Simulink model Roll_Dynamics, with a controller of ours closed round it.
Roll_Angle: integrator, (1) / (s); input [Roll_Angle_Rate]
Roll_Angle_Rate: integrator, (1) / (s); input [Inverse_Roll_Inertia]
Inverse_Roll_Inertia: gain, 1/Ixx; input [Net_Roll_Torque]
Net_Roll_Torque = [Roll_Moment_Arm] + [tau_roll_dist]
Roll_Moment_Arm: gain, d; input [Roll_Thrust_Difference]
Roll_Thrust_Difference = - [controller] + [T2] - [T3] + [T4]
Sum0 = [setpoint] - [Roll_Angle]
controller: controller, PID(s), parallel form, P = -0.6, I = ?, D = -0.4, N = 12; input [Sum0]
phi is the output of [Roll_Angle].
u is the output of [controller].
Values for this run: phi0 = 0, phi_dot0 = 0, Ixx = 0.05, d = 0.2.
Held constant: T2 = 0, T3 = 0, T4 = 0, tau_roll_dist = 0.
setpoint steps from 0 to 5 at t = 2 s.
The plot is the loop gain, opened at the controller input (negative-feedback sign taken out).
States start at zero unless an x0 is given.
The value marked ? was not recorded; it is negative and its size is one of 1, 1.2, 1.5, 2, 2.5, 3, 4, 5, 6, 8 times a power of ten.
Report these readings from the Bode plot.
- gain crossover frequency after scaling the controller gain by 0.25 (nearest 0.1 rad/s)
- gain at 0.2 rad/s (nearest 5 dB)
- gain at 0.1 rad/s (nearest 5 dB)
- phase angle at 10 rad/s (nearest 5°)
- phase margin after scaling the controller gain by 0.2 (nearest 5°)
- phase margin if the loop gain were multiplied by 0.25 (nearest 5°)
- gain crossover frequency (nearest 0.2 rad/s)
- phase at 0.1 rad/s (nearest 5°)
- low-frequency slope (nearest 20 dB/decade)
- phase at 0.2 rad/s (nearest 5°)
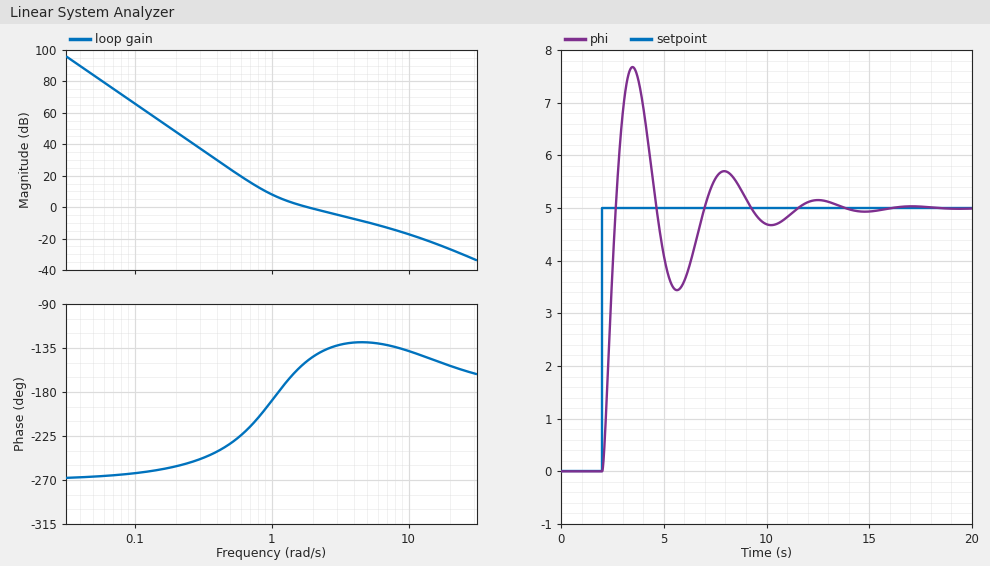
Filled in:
0.8 rad/s
50 dB
65 dB
-140°
-30°
-25°
1.8 rad/s
-265°
-60 dB/decade
-255°
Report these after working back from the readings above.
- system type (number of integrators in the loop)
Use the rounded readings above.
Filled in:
3
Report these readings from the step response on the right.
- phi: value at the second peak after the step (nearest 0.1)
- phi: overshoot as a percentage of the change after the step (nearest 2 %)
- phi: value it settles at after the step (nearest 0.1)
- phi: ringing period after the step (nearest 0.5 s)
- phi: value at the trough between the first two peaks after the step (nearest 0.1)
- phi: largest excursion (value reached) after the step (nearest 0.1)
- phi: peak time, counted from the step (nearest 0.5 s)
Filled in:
5.7
54 %
5.0
4.5 s
3.4
7.7
1.5 s
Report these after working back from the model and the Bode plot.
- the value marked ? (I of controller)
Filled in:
-0.5
